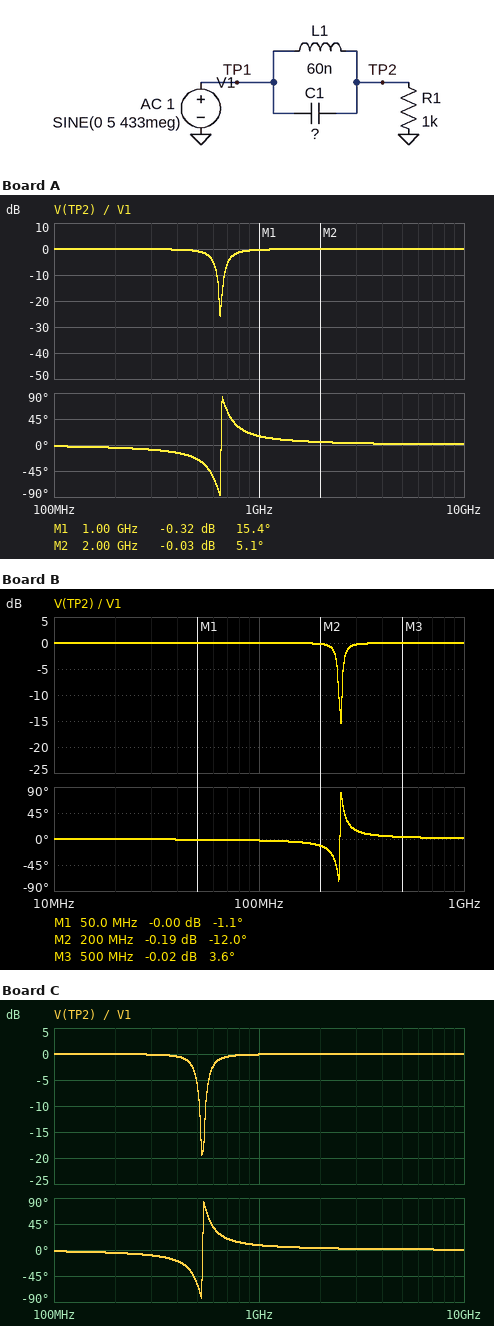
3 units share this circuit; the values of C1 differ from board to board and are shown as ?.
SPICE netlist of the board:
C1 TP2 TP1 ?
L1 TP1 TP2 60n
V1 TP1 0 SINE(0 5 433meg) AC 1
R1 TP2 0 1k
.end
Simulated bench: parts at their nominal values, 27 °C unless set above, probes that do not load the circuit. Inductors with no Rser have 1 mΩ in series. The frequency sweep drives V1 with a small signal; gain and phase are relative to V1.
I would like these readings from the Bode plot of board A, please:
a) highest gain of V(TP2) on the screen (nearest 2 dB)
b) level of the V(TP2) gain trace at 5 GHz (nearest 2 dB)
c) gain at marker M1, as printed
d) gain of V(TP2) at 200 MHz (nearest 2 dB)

0 dB
0 dB
-0.32 dB
0 dB
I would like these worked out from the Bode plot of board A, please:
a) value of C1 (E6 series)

1 pF
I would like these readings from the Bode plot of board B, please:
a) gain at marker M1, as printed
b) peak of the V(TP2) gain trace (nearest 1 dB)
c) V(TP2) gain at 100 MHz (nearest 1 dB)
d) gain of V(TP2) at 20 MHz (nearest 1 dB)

-0.00 dB
0 dB
0 dB
0 dB
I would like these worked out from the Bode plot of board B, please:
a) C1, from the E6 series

6.8 pF
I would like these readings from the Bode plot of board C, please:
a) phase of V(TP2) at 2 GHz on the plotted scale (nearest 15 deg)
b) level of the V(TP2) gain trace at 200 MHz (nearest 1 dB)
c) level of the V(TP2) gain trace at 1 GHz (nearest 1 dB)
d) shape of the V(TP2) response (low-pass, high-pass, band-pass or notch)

0 deg
0 dB
0 dB
notch
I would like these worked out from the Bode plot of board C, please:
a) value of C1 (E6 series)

1.5 pF
